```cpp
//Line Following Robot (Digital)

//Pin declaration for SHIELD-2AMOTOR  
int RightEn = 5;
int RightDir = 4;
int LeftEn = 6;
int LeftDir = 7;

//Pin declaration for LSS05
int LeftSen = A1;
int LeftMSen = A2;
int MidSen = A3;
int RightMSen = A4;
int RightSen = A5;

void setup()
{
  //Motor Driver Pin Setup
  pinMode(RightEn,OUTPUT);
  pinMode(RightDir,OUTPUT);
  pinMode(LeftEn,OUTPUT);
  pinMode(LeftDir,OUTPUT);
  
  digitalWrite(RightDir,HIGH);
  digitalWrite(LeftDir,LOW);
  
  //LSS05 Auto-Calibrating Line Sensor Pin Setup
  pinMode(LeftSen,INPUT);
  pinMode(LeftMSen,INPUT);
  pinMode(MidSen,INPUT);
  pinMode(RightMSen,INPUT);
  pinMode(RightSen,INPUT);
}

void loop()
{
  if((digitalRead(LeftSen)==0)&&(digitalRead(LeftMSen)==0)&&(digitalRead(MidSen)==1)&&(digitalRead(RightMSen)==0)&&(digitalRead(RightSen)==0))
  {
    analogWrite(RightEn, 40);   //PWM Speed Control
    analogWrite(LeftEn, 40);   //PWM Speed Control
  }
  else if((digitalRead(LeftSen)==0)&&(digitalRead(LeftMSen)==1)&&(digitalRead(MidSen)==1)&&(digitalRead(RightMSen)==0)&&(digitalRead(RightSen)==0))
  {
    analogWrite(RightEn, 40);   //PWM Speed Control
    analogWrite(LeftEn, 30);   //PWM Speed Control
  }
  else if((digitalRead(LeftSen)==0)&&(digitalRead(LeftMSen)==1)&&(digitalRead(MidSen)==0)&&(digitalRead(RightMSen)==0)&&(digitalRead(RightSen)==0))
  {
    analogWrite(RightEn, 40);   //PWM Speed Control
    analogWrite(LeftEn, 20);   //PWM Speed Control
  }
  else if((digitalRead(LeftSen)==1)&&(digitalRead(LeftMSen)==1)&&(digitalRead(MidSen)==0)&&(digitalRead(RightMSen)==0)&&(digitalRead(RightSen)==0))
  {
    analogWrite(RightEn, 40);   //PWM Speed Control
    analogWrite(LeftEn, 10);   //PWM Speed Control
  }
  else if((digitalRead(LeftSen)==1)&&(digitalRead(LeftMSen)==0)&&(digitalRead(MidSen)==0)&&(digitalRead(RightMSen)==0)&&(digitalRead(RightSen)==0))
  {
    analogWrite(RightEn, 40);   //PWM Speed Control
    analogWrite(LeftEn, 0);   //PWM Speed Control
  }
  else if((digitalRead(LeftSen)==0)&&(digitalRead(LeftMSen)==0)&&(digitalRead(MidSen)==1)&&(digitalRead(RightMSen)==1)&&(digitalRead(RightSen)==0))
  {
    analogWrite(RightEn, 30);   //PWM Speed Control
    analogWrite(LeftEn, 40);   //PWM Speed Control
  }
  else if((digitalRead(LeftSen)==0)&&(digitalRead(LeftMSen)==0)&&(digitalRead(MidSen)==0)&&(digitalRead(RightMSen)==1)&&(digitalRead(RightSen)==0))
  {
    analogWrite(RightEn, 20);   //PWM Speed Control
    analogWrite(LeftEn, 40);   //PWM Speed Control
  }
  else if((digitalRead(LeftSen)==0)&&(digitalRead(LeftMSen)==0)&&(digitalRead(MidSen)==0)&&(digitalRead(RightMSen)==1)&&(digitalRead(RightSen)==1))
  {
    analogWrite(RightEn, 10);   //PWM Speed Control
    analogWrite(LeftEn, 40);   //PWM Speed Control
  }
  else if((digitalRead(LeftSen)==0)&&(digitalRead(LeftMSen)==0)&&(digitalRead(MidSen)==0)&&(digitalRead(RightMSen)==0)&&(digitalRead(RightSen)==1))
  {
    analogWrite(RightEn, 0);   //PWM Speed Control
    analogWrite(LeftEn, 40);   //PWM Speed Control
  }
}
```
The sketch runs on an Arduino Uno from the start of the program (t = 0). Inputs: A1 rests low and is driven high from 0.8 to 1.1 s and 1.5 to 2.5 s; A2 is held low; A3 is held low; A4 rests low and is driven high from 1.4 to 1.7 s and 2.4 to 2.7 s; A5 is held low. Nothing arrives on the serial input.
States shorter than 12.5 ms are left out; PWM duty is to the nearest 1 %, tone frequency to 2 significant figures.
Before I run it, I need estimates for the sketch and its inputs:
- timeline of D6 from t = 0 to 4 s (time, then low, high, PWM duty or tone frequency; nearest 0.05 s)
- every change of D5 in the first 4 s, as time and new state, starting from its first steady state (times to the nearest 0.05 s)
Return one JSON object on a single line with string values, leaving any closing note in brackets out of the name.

{"timeline of D6 from t = 0 to 4 s": "0 s low; 1.4 s PWM 16 %; 1.7 s low; 2.5 s PWM 16 %", "every change of D5 in the first 4 s, as time and new state, starting from its first steady state": "0 s low; 0.8 s PWM 16 %; 1.4 s PWM 8 %; 1.7 s PWM 16 %; 2.5 s PWM 8 %"}
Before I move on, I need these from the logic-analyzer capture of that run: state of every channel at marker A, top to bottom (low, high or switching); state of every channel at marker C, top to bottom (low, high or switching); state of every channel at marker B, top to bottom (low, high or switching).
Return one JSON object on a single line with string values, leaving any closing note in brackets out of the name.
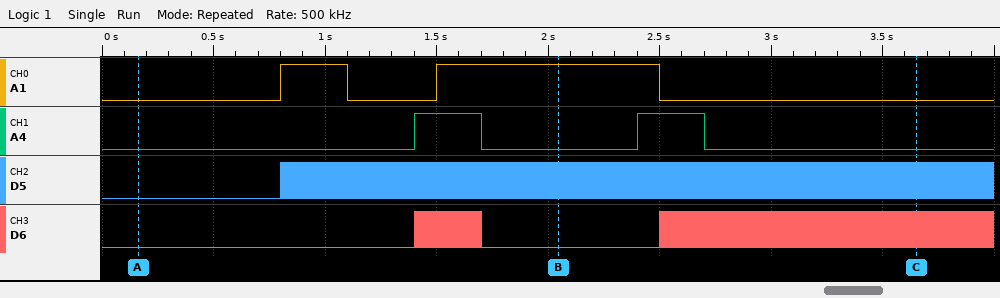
{"state of every channel at marker A, top to bottom": "A1 low, A4 low, D5 low, D6 low", "state of every channel at marker C, top to bottom": "A1 low, A4 low, D5 switching, D6 switching", "state of every channel at marker B, top to bottom": "A1 high, A4 low, D5 switching, D6 low"}
